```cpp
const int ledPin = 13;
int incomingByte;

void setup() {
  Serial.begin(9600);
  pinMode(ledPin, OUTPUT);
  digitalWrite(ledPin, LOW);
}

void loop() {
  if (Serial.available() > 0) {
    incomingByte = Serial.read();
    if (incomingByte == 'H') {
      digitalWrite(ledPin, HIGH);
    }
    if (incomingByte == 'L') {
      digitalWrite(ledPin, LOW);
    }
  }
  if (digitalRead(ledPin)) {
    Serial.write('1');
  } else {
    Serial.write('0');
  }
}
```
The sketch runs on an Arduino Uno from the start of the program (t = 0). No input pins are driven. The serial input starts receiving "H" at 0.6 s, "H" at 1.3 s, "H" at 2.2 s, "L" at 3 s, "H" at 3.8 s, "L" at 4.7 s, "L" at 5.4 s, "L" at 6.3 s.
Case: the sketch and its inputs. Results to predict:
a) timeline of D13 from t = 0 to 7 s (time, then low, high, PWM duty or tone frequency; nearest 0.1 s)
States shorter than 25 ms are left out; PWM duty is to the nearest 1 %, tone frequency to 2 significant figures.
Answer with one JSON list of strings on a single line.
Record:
["0 s low; 0.6 s high; 3 s low; 3.8 s high; 4.7 s low"]
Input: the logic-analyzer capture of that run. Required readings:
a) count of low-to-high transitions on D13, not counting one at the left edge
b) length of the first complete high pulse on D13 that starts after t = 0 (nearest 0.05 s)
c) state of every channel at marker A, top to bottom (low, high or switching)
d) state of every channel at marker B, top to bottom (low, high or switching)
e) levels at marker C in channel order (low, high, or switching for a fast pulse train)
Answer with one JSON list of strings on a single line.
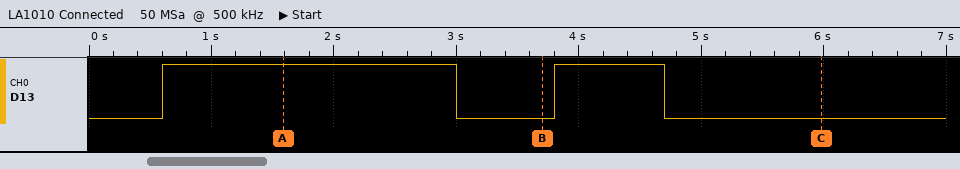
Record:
["2", "2.40 s", "D13 high", "D13 low", "D13 low"]
